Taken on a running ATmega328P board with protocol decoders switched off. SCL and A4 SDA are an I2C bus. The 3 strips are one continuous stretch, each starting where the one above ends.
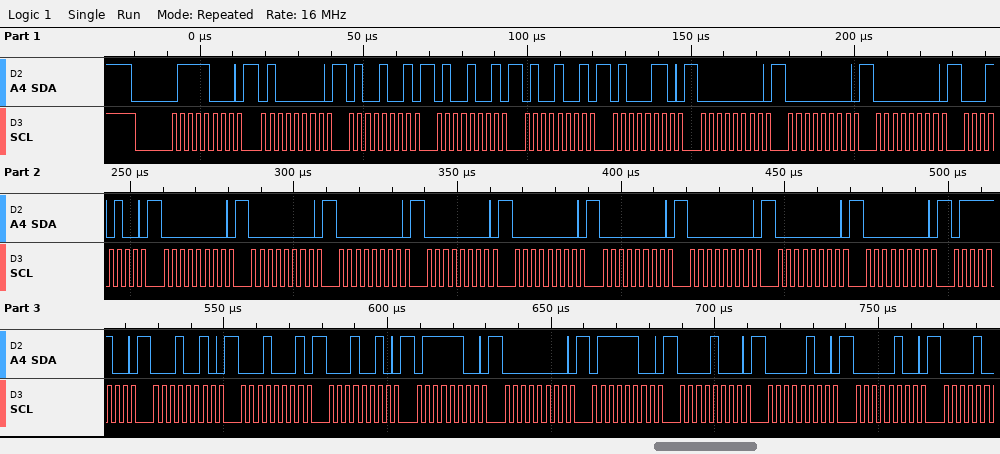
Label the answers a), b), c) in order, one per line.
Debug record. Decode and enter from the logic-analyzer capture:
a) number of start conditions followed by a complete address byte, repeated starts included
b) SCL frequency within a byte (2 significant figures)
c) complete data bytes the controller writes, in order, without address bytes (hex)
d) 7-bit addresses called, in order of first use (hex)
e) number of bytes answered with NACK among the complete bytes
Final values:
a) 1
b) 400 kHz
c) 40 49 49 49 46 00 00 00 14 00 00 00 00 00 00 00 00 00 7C 12 11 12 7C 00 7C 08 04 04
d) 0x3C
e) 0
